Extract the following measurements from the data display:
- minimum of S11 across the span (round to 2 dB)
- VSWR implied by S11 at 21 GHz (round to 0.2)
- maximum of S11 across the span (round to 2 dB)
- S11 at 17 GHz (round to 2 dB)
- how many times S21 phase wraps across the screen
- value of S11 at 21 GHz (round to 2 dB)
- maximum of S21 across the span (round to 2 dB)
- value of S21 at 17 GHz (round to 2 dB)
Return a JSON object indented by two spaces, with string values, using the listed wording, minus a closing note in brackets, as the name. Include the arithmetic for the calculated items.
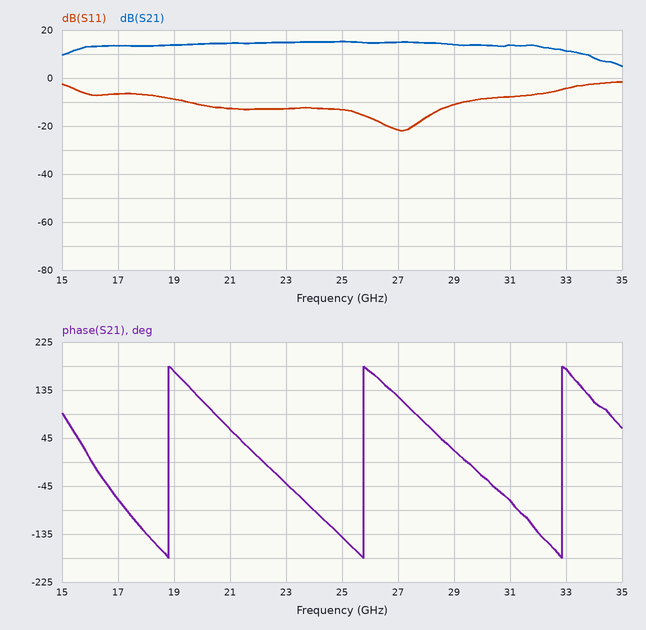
{
  "minimum of S11 across the span": "-22 dB",
  "VSWR implied by S11 at 21 GHz": "|Γ| = 10^(-12/20) = 0.2512; VSWR = (1 + 0.2512)/(1 − 0.2512) ≈ 1.67, so 1.6 to the nearest 0.2",
  "maximum of S11 across the span": "-2 dB",
  "S11 at 17 GHz": "-6 dB",
  "how many times S21 phase wraps across the screen": "3",
  "value of S11 at 21 GHz": "-12 dB",
  "maximum of S21 across the span": "16 dB",
  "value of S21 at 17 GHz": "14 dB"
}
